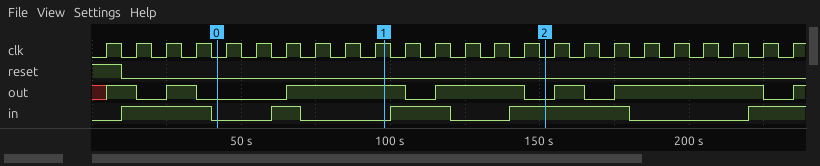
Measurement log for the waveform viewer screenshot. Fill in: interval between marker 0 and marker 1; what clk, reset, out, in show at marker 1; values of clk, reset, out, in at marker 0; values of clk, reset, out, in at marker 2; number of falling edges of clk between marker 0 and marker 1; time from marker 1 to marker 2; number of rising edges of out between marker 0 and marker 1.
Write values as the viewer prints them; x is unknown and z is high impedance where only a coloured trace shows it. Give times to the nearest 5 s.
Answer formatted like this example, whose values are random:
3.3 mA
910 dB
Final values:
55 s
clk=1, reset=0, out=1, in=0
clk=0, reset=0, out=0, in=0
clk=0, reset=0, out=0, in=1
5
55 s
1
